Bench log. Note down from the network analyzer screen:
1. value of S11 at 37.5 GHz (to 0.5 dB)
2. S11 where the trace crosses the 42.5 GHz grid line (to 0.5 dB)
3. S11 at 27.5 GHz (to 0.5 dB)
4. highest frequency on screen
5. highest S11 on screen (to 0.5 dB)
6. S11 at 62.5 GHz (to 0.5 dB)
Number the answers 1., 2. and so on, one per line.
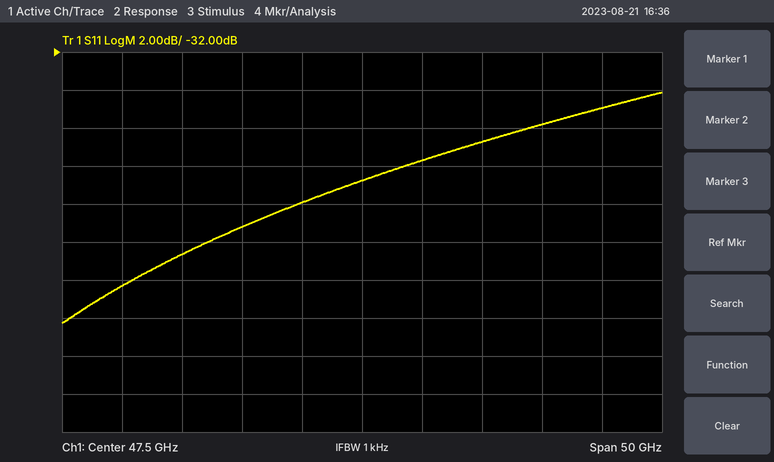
1. -41.0 dB
2. -40.0 dB
3. -44.5 dB
4. 72.5 GHz
5. -34.0 dB
6. -36.0 dB
